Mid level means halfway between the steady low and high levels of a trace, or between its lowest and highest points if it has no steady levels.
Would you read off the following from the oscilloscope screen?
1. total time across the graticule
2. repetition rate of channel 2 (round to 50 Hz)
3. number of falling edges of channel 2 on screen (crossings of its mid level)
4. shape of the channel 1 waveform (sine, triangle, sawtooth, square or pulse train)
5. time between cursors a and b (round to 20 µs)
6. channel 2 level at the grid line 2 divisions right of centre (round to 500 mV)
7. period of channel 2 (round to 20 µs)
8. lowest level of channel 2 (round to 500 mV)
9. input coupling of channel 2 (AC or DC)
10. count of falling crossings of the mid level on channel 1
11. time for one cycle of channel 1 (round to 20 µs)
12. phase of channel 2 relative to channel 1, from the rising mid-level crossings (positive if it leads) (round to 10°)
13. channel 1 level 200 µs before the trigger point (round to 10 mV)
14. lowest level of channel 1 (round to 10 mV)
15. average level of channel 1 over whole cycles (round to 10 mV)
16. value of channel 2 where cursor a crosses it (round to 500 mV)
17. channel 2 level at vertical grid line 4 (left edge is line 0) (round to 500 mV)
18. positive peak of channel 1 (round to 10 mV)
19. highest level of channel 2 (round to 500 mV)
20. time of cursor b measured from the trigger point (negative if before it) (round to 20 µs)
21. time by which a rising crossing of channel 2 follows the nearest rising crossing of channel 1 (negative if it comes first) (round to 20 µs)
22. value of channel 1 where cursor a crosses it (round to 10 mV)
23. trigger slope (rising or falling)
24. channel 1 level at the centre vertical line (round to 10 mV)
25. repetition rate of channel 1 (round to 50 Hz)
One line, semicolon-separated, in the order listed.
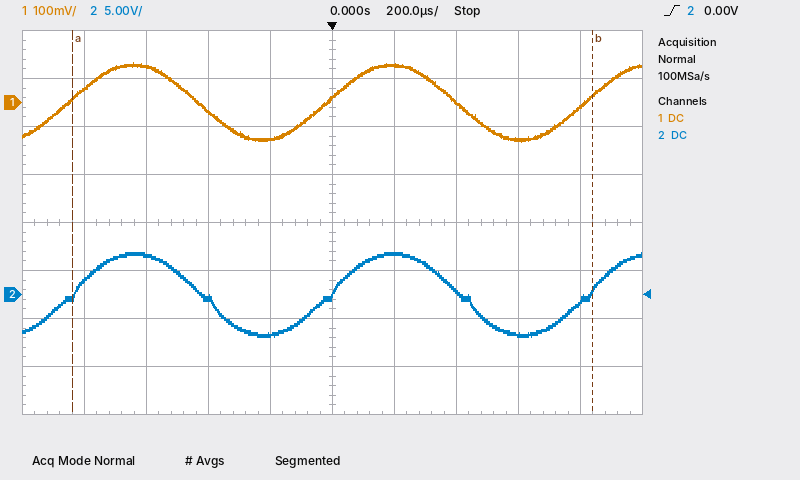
2 ms; 1.20 kHz; 2; sine; 1.68 ms; 500 mV; 840 µs; -4.5 V; DC; 2; 840 µs; -10°; -80 mV; -80 mV; 0 mV; 0.0 V; -4.0 V; 80 mV; 4.5 V; +840 µs; +20 µs; 10 mV; rising; 10 mV; 1.20 kHz
